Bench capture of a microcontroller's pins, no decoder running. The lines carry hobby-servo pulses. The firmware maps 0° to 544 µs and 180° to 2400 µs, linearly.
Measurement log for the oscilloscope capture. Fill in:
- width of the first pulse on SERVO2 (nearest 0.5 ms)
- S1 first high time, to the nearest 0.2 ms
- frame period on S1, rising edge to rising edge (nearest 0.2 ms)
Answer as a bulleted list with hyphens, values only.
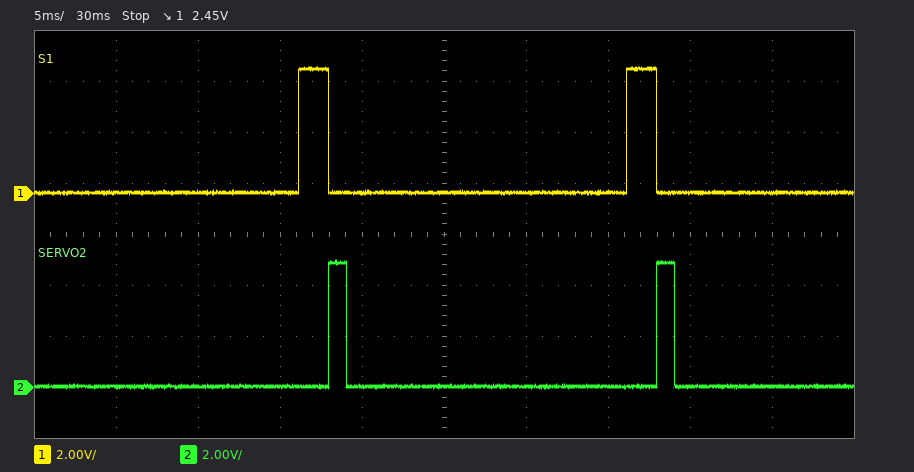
- 1.0 ms
- 1.8 ms
- 20.0 ms
